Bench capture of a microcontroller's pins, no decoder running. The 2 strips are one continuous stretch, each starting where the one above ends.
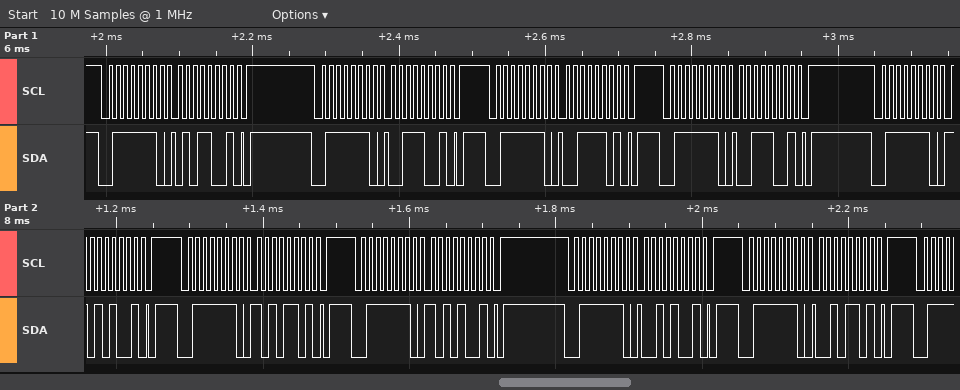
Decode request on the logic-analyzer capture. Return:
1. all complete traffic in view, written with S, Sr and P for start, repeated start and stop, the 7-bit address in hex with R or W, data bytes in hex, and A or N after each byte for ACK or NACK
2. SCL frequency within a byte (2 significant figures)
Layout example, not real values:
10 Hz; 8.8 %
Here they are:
S 3FW A 59 A P S 3FW A 39 A P S 3FW A 3D A P S 3FW A 39 A P S 3FW A A9 A P S 3FW A AD A P S 3FW A A9 A P S 3FW A 29 A P S 3FW A 2D A P; 100 kHz
